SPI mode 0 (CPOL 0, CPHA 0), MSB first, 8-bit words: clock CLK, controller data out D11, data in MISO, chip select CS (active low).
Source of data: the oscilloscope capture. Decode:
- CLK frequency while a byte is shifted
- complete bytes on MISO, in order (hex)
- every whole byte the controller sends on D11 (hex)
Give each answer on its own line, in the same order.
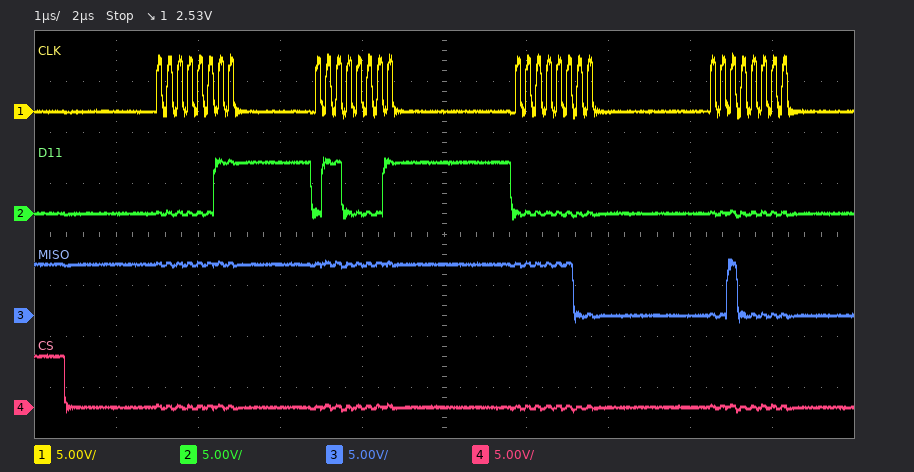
8 MHz
FF FF FC 20
03 61 00 00
